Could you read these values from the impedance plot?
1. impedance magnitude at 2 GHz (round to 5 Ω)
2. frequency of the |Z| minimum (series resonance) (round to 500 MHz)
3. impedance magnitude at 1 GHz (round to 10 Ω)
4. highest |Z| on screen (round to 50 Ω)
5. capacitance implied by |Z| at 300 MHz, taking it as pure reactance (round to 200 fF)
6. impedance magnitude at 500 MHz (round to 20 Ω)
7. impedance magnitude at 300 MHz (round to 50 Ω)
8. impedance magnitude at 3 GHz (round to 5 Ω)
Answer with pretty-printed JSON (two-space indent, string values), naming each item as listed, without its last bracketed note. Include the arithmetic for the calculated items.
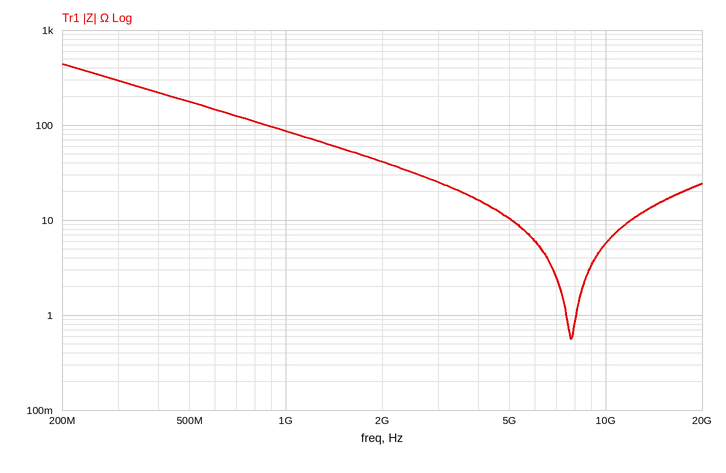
{
  "impedance magnitude at 2 GHz": "40 Ω",
  "frequency of the |Z| minimum (series resonance)": "8.0 GHz",
  "impedance magnitude at 1 GHz": "90 Ω",
  "highest |Z| on screen": "450 Ω",
  "capacitance implied by |Z| at 300 MHz, taking it as pure reactance": "C = 1/(2π × 300 MHz × 300 Ω) ≈ 1.8 pF",
  "impedance magnitude at 500 MHz": "180 Ω",
  "impedance magnitude at 300 MHz": "300 Ω",
  "impedance magnitude at 3 GHz": "25 Ω"
}
